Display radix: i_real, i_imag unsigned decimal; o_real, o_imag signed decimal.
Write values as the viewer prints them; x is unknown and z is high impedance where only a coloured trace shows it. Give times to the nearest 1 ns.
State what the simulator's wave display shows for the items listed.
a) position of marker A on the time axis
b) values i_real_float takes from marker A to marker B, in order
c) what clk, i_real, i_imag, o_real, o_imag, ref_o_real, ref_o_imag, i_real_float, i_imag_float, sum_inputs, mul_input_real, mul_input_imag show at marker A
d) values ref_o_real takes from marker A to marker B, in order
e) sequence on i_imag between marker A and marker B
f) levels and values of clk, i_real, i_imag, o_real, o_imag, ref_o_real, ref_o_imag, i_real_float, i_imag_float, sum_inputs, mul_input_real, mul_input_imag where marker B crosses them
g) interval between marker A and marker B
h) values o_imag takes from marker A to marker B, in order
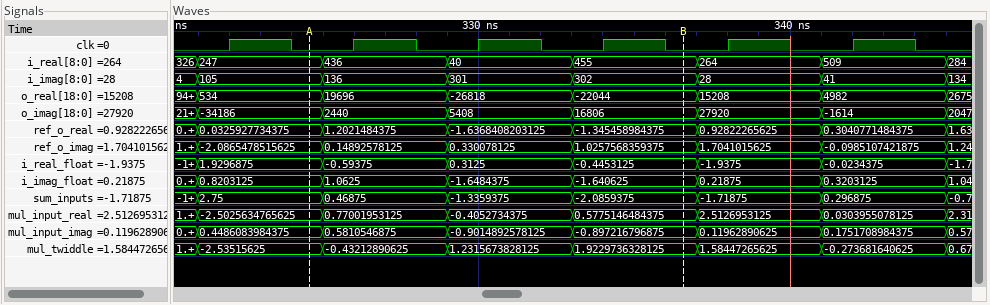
325 ns
1.9296875, -0.59375, 0.3125, -0.4453125
clk=0, i_real=247, i_imag=105, o_real=534, o_imag=-34186, ref_o_real=0.0325927734375, ref_o_imag=-2.0865478515625, i_real_float=1.9296875, i_imag_float=0.8203125, sum_inputs=2.75, mul_input_real=-2.5025634765625, mul_input_imag=0.4486083984375
0.0325927734375, 1.2021484375, -1.6368408203125, -1.345458984375
105, 136, 301, 302
clk=0, i_real=455, i_imag=302, o_real=-22044, o_imag=16806, ref_o_real=-1.345458984375, ref_o_imag=1.0257568359375, i_real_float=-0.4453125, i_imag_float=-1.640625, sum_inputs=-2.0859375, mul_input_real=0.5775146484375, mul_input_imag=-0.897216796875
12 ns
-34186, 2440, 5408, 16806
